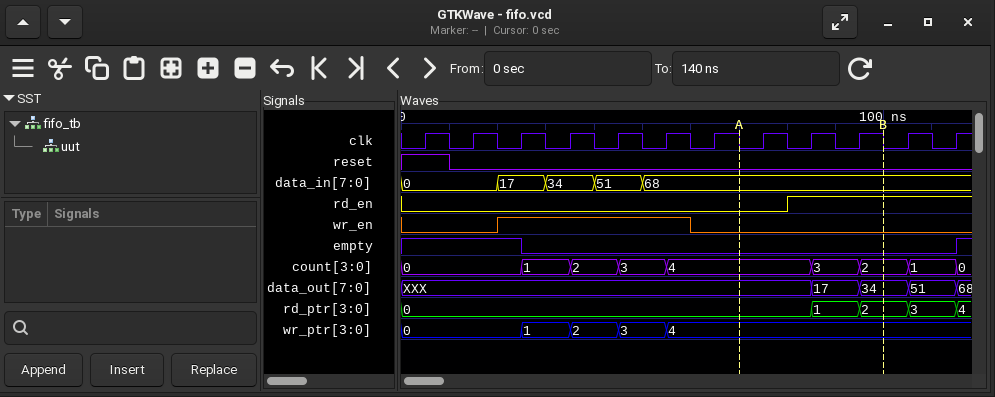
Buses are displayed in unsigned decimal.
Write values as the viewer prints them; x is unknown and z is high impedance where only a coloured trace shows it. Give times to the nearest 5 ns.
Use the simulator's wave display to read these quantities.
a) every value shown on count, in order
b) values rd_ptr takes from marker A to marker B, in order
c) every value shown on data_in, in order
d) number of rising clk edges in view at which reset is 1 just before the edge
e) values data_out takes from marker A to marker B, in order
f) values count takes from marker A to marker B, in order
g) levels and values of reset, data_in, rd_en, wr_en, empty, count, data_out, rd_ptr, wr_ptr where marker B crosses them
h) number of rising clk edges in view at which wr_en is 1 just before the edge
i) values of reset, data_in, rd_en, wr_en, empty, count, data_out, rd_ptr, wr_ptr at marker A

0, 1, 2, 3, 4, 3, 2, 1, 0
0, 1, 2
0, 17, 34, 51, 68
1
XXX, 17, 34
4, 3, 2
reset=0, data_in=68, rd_en=1, wr_en=0, empty=0, count=2, data_out=34, rd_ptr=2, wr_ptr=4
4
reset=0, data_in=68, rd_en=0, wr_en=0, empty=0, count=4, data_out=XXX, rd_ptr=0, wr_ptr=4
